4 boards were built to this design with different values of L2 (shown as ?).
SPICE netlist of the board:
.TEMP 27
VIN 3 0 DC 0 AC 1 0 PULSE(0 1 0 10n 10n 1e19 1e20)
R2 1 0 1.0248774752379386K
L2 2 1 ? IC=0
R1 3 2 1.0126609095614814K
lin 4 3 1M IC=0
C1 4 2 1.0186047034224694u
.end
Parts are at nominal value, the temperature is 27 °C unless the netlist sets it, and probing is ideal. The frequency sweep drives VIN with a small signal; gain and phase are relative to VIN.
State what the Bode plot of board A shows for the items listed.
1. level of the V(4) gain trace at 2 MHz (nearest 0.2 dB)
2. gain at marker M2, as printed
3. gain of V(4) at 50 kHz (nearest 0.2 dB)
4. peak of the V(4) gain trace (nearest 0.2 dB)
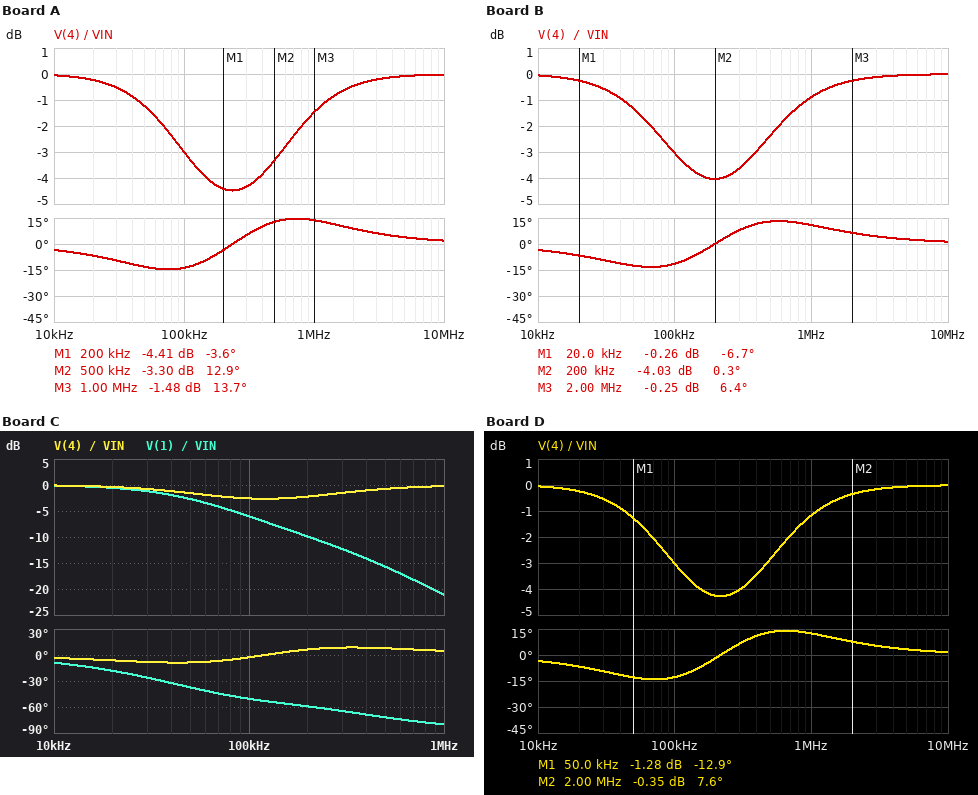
-0.4 dB
-3.30 dB
-1.2 dB
0 dB
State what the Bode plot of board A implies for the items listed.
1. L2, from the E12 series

470 µH
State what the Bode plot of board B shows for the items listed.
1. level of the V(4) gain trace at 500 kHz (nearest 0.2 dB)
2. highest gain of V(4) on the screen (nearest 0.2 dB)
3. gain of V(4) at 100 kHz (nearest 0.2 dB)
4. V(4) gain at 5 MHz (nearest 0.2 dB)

-2.4 dB
0 dB
-3.0 dB
0 dB
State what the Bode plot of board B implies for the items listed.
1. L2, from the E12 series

680 µH
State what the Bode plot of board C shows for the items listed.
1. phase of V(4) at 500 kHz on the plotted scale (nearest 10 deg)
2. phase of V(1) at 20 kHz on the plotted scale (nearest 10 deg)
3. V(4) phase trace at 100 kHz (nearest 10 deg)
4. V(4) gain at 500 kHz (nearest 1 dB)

10 deg
-20 deg
0 deg
-1 dB
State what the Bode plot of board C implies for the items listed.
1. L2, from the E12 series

1.8 mH
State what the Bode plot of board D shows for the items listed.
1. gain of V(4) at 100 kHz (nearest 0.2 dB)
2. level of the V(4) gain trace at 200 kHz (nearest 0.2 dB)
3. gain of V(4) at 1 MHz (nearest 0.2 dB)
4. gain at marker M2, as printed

-3.0 dB
-4.2 dB
-1.2 dB
-0.35 dB
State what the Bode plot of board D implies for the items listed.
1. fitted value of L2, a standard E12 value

560 µH
